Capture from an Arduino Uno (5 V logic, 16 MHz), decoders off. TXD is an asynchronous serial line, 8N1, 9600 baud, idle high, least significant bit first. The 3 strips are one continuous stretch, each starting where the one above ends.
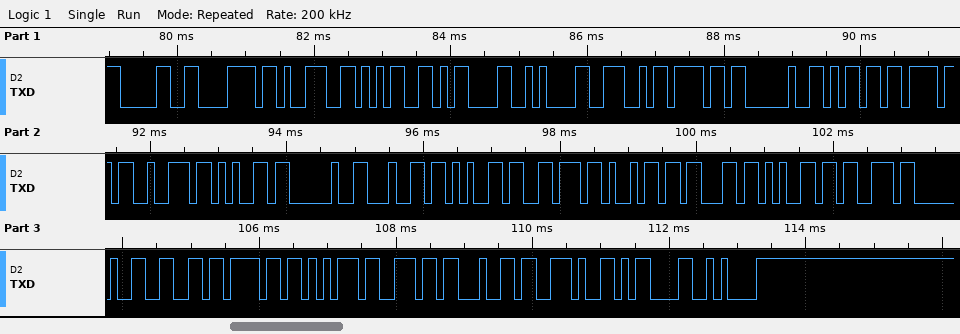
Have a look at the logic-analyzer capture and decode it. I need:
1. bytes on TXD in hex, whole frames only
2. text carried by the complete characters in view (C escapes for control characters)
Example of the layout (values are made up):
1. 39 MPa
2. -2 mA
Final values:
1. 30 78 39 35 0D 0A 4E 6F 20 6D 6F 72 65 20 64 65 76 69 63 65 73 20 66 6F 75 6E 64 2E 0D 0A
2. "0x95\r\nNo more devices found.\r\n"
